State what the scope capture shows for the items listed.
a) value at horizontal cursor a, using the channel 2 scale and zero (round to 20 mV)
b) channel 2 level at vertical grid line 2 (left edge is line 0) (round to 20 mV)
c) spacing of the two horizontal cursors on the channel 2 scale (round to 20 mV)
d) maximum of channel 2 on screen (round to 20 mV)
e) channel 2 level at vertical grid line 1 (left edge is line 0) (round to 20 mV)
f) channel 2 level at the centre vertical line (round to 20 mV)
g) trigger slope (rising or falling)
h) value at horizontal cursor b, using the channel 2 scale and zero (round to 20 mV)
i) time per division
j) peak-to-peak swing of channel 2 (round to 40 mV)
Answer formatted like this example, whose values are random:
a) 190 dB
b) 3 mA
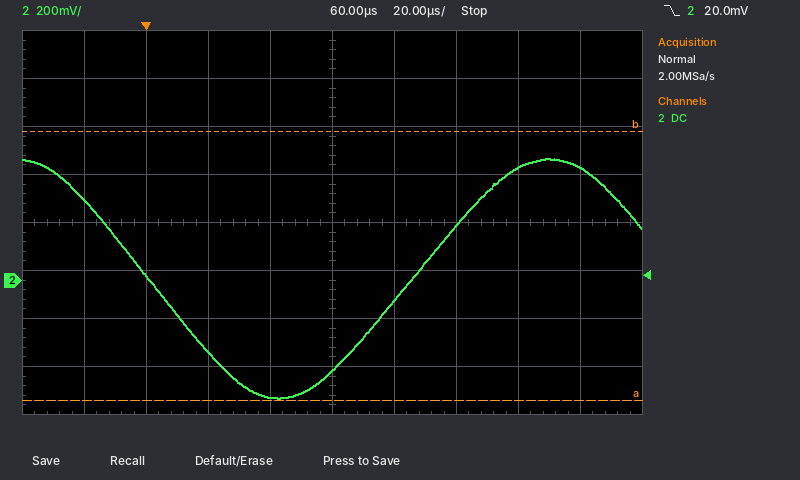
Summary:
a) -500 mV
b) 20 mV
c) 1.12 V
d) 500 mV
e) 340 mV
f) -380 mV
g) falling
h) 620 mV
i) 20 µs
j) 1.00 V
